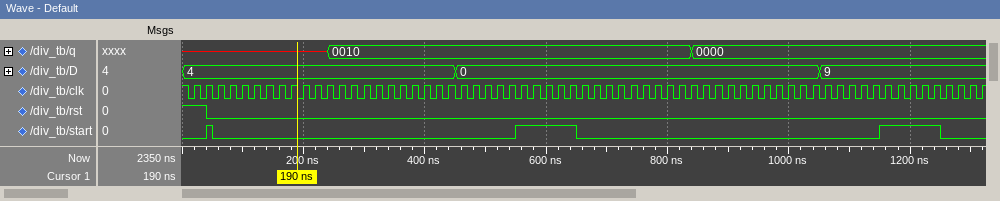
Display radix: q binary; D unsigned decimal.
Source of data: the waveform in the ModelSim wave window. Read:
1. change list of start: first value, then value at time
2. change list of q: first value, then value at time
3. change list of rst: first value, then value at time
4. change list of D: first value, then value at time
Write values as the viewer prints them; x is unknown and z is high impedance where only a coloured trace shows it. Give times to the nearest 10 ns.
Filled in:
0, 1 at 40 ns, 0 at 50 ns, 1 at 550 ns, 0 at 650 ns, 1 at 1150 ns, 0 at 1250 ns
x, 0010 at 240 ns, 0000 at 840 ns
1, 0 at 40 ns
4, 0 at 450 ns, 9 at 1050 ns
